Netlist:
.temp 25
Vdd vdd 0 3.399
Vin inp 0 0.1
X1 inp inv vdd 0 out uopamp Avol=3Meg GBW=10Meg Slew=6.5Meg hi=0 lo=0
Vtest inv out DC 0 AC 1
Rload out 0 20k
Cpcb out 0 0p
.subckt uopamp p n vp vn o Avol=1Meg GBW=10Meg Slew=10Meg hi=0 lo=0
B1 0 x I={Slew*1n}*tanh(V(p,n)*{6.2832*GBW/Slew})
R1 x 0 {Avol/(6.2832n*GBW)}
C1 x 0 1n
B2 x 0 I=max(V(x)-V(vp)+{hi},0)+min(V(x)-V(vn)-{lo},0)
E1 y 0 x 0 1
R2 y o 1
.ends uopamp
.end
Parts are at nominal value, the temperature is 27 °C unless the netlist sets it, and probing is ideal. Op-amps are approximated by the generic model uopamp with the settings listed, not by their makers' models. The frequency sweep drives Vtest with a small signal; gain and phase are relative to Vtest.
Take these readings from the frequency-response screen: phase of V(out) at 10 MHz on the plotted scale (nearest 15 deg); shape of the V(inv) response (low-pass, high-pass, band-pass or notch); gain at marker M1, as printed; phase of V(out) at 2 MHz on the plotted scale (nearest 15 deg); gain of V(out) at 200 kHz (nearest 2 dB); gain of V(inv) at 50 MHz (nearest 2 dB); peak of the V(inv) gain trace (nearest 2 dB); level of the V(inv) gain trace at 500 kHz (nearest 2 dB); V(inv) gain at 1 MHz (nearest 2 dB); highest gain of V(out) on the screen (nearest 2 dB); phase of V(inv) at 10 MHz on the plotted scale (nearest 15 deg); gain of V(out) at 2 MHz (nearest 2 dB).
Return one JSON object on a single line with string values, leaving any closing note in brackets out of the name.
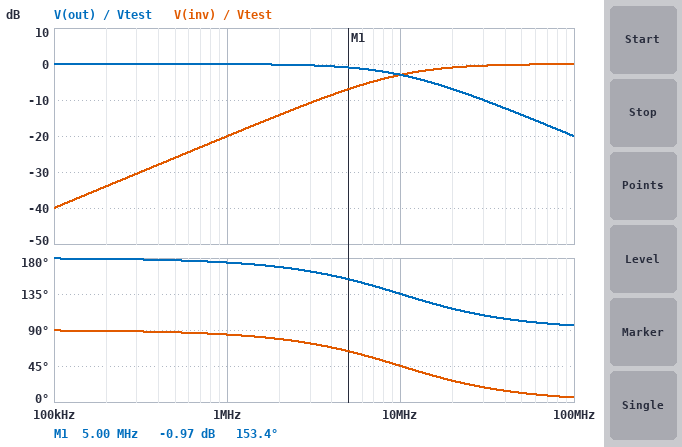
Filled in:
{"phase of V(out) at 10 MHz on the plotted scale": "135 deg", "shape of the V(inv) response": "high-pass", "gain at marker M1, as printed": "-0.97 dB", "phase of V(out) at 2 MHz on the plotted scale": "165 deg", "gain of V(out) at 200 kHz": "0 dB", "gain of V(inv) at 50 MHz": "0 dB", "peak of the V(inv) gain trace": "0 dB", "level of the V(inv) gain trace at 500 kHz": "-26 dB", "V(inv) gain at 1 MHz": "-20 dB", "highest gain of V(out) on the screen": "0 dB", "phase of V(inv) at 10 MHz on the plotted scale": "45 deg", "gain of V(out) at 2 MHz": "0 dB"}
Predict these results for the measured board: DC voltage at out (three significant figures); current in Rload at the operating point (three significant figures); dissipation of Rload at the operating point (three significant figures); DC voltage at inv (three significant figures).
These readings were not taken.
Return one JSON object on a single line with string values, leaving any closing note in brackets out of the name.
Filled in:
{"DC voltage at out": "100 mV", "current in Rload at the operating point": "5.00 µA", "dissipation of Rload at the operating point": "500 nW", "DC voltage at inv": "100 mV"}
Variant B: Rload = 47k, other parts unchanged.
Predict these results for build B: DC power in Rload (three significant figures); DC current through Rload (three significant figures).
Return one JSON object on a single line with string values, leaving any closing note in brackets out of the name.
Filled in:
{"DC power in Rload": "213 nW", "DC current through Rload": "2.13 µA"}
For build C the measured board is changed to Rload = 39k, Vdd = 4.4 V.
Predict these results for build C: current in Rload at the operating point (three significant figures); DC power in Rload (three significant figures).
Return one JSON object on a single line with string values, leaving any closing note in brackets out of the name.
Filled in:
{"current in Rload at the operating point": "2.56 µA", "DC power in Rload": "256 nW"}
